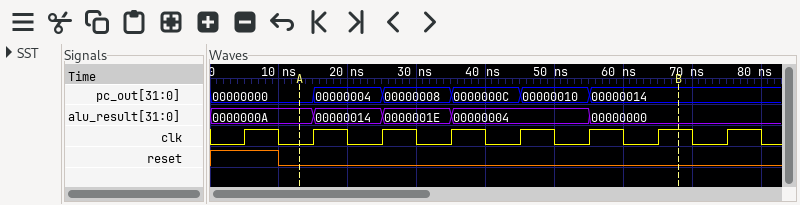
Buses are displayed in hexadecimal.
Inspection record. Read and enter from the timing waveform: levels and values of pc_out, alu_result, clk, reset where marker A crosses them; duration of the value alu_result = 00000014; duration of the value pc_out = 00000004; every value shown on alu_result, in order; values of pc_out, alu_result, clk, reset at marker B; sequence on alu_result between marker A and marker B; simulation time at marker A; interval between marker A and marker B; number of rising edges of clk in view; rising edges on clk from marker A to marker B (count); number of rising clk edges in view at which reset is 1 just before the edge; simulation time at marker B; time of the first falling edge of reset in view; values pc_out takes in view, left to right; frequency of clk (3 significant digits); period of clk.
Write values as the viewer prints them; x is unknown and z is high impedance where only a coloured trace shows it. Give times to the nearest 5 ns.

pc_out=00000000, alu_result=0000000A, clk=0, reset=0
10 ns
10 ns
0000000A, 00000014, 0000001E, 00000004, 00000000
pc_out=00000014, alu_result=00000000, clk=1, reset=0
0000000A, 00000014, 0000001E, 00000004, 00000000
15 ns
55 ns
8
6
1
70 ns
10 ns
00000000, 00000004, 00000008, 0000000C, 00000010, 00000014
100 MHz
10 ns
